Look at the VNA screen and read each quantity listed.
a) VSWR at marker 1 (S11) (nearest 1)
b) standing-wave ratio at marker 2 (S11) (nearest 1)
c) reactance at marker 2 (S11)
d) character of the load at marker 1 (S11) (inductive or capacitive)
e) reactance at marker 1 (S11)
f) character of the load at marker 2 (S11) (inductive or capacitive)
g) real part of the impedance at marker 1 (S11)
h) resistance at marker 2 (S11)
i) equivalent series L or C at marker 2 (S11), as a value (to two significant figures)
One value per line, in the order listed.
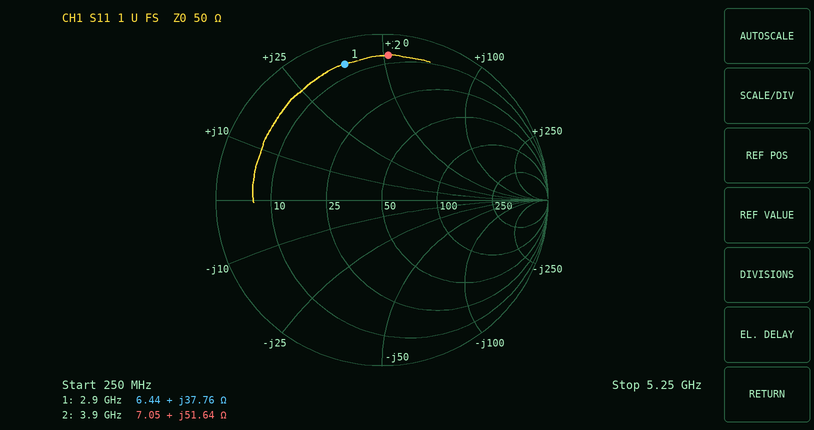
12
15
+51.64 Ω
inductive
+37.76 Ω
inductive
6.44 Ω
7.05 Ω
2.1 nH
